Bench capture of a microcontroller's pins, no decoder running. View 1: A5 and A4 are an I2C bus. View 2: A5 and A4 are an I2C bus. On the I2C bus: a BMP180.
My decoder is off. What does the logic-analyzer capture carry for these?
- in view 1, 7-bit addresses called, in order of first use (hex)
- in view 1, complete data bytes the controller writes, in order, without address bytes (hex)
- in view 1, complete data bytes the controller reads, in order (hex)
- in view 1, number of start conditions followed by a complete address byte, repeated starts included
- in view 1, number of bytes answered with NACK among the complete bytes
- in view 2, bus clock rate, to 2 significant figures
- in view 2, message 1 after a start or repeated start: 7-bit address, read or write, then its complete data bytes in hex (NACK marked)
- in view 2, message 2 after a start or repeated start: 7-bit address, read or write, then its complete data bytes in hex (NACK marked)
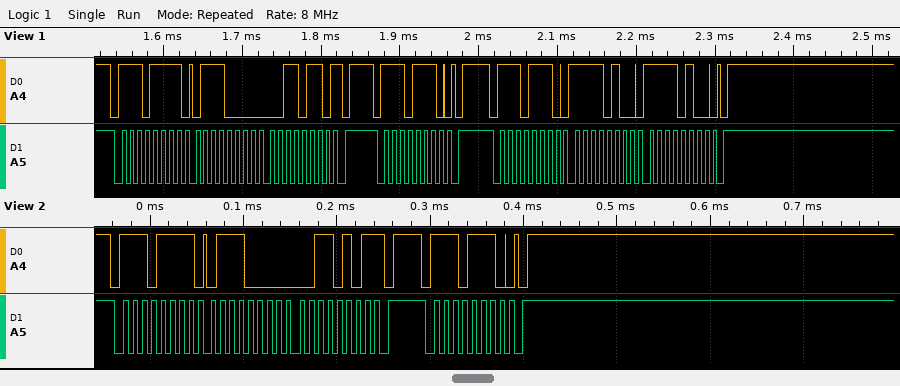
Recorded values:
0x77
F4 F4
70 36
3
1
100 kHz
0x77 read: 70 35 NACK
0x77 write
